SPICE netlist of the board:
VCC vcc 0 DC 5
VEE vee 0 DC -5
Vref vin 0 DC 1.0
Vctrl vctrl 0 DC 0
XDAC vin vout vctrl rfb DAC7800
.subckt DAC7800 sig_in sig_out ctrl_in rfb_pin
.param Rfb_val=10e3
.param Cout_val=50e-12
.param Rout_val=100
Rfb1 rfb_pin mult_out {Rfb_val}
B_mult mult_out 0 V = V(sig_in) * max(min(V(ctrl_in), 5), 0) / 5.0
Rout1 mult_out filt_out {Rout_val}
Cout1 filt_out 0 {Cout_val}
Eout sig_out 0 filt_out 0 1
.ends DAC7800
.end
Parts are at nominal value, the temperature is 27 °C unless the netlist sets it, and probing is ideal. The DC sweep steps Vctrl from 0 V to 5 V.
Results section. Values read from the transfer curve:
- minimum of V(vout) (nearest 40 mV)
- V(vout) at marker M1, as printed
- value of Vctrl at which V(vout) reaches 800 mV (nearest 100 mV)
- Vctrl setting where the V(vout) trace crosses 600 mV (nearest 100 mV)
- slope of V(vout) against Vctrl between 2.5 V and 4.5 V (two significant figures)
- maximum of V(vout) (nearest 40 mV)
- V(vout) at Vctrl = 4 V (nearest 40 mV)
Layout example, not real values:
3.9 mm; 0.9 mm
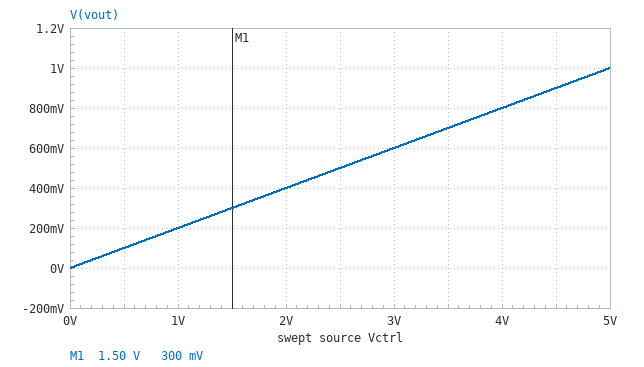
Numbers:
0 V; 300 mV; 4.0 V; 3.0 V; 0.20 V/V; 1.00 V; 800 mV
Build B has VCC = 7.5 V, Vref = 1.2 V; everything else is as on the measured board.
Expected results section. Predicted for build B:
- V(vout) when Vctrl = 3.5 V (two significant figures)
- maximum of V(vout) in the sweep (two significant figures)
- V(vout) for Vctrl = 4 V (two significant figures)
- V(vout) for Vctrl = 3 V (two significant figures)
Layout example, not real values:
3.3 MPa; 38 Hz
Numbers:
840 mV; 1.2 V; 960 mV; 720 mV
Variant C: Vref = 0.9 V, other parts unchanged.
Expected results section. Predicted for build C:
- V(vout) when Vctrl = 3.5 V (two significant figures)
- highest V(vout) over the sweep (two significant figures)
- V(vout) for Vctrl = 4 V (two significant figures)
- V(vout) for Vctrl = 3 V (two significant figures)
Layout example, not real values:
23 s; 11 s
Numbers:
630 mV; 900 mV; 720 mV; 540 mV
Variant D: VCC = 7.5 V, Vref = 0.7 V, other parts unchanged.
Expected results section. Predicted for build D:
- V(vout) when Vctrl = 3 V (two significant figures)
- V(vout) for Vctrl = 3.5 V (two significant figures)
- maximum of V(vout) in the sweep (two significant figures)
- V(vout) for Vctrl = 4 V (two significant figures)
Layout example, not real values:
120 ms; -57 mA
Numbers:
420 mV; 490 mV; 700 mV; 560 mV
